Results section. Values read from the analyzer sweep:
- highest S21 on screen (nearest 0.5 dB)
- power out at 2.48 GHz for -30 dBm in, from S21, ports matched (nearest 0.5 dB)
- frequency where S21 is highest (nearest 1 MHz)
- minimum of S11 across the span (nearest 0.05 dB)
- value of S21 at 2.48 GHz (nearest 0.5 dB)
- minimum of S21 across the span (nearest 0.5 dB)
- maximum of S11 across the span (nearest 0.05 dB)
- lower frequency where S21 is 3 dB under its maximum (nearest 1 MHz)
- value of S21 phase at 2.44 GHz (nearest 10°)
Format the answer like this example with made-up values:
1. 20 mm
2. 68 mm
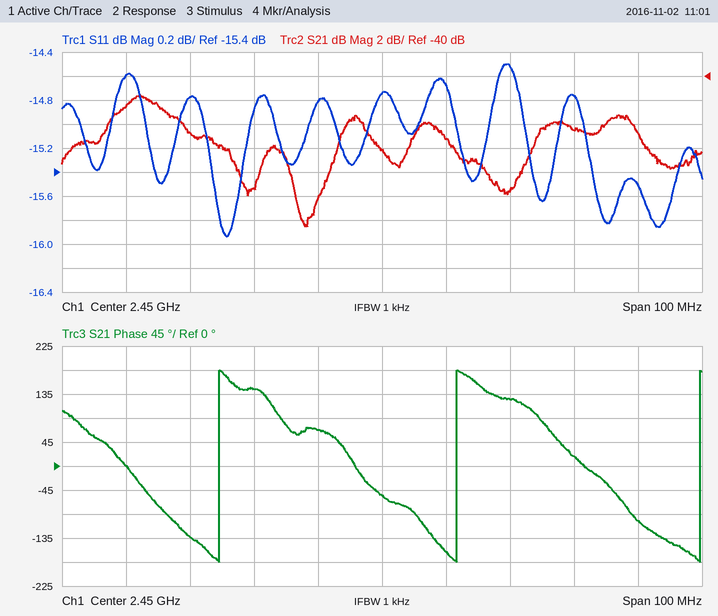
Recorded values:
1. -41.5 dB
2. -74.5 dBm
3. 2.412 GHz
4. -15.95 dB
5. -44.5 dB
6. -52.5 dB
7. -14.50 dB
8. 2.407 GHz
9. 70°
